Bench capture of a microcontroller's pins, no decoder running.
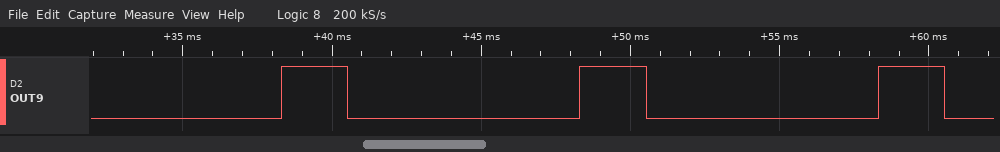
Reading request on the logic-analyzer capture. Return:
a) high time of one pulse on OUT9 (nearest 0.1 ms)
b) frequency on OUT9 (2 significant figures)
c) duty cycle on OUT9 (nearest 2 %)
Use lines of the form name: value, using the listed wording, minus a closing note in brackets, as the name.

high time of one pulse on OUT9: 2.2 ms
frequency on OUT9: 100 Hz
duty cycle on OUT9: 22 %
